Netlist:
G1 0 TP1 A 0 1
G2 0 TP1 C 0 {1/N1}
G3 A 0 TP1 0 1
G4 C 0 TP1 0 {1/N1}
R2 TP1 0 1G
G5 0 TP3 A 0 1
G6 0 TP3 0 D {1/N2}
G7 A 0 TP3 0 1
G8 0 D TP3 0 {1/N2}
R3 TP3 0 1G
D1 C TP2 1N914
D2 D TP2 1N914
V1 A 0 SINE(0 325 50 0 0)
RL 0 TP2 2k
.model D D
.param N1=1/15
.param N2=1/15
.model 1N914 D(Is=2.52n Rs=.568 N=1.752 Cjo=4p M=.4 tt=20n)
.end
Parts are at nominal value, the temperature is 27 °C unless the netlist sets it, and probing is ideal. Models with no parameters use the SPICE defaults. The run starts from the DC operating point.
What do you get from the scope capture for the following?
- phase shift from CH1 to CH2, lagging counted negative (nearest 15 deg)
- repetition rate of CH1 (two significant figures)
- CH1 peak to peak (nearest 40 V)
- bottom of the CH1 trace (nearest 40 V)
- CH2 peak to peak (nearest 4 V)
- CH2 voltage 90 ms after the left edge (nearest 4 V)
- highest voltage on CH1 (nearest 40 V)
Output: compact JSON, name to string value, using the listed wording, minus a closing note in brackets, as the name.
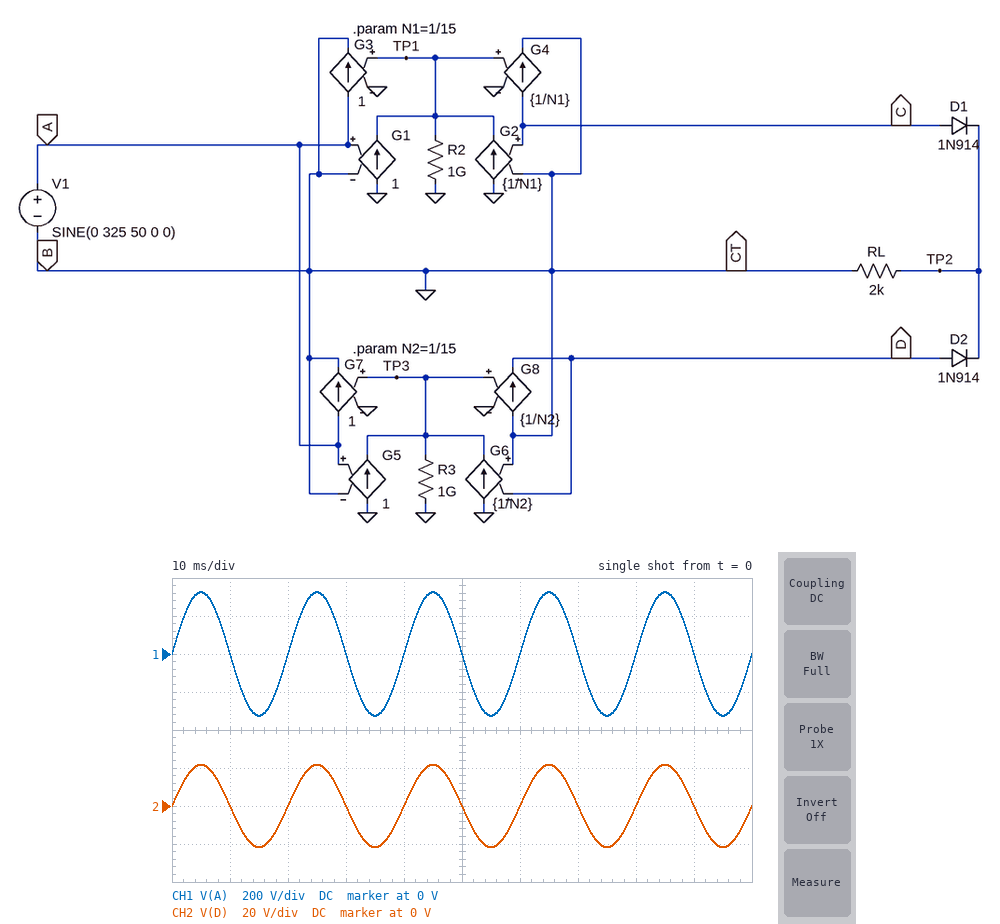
{"phase shift from CH1 to CH2, lagging counted negative": "0 deg", "repetition rate of CH1": "50 Hz", "CH1 peak to peak": "640 V", "bottom of the CH1 trace": "-320 V", "CH2 peak to peak": "44 V", "CH2 voltage 90 ms after the left edge": "0 V", "highest voltage on CH1": "320 V"}
